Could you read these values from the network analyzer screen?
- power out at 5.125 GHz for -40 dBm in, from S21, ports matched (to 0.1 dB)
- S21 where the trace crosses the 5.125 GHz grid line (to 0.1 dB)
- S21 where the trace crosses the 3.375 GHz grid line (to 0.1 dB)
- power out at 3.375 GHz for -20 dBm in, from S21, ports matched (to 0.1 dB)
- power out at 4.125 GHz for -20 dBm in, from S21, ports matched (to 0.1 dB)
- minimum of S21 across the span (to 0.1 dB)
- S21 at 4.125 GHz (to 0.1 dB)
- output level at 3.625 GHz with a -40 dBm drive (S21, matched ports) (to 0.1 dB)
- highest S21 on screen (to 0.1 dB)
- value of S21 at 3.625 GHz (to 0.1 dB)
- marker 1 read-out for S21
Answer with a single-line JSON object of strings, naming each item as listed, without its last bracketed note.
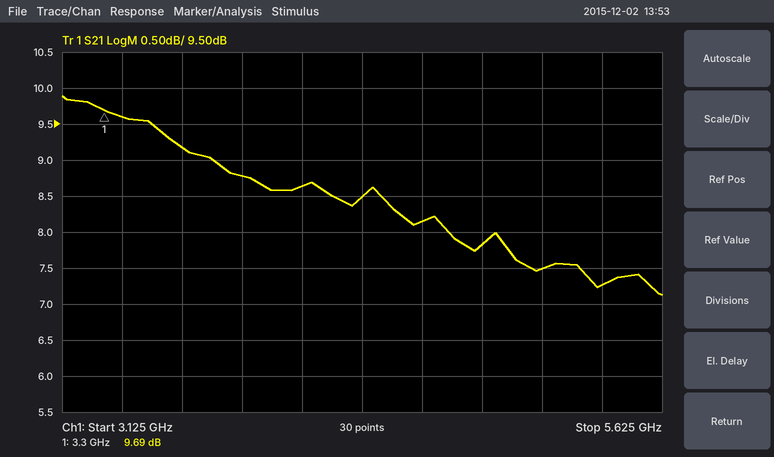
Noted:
{"power out at 5.125 GHz for -40 dBm in, from S21, ports matched": "-32.5 dBm", "S21 where the trace crosses the 5.125 GHz grid line": "7.5 dB", "S21 where the trace crosses the 3.375 GHz grid line": "9.6 dB", "power out at 3.375 GHz for -20 dBm in, from S21, ports matched": "-10.4 dBm", "power out at 4.125 GHz for -20 dBm in, from S21, ports matched": "-11.4 dBm", "minimum of S21 across the span": "7.1 dB", "S21 at 4.125 GHz": "8.6 dB", "output level at 3.625 GHz with a -40 dBm drive (S21, matched ports)": "-30.8 dBm", "highest S21 on screen": "9.9 dB", "value of S21 at 3.625 GHz": "9.2 dB", "marker 1 read-out for S21": "9.69 dB"}
